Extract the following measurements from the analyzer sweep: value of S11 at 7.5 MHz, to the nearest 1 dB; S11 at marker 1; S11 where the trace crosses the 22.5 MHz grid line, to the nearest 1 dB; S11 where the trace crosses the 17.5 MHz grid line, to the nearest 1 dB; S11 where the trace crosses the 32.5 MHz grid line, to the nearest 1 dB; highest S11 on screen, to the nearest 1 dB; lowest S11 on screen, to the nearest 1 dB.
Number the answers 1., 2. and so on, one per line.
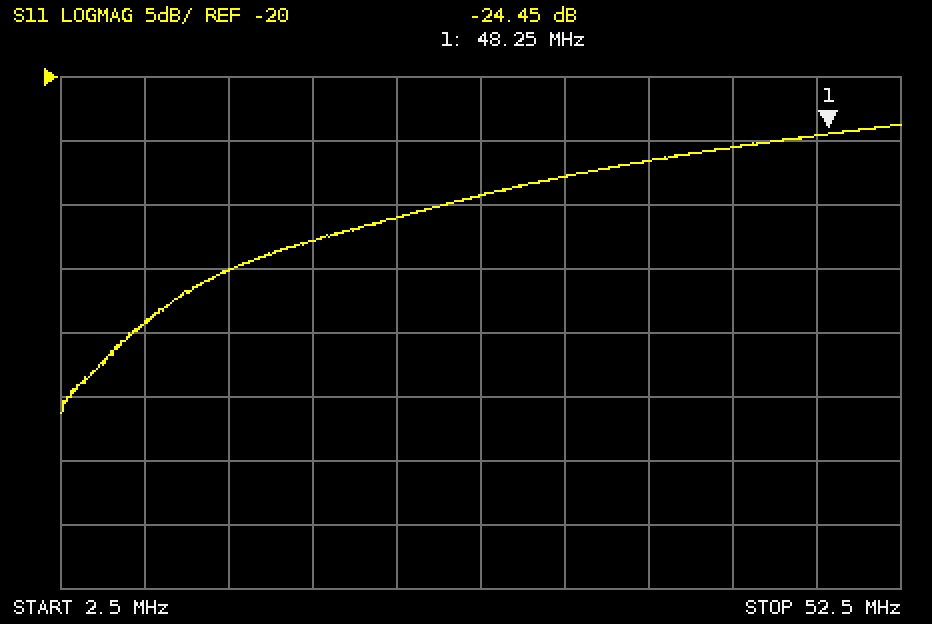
1. -39 dB
2. -24.45 dB
3. -31 dB
4. -33 dB
5. -28 dB
6. -24 dB
7. -46 dB
